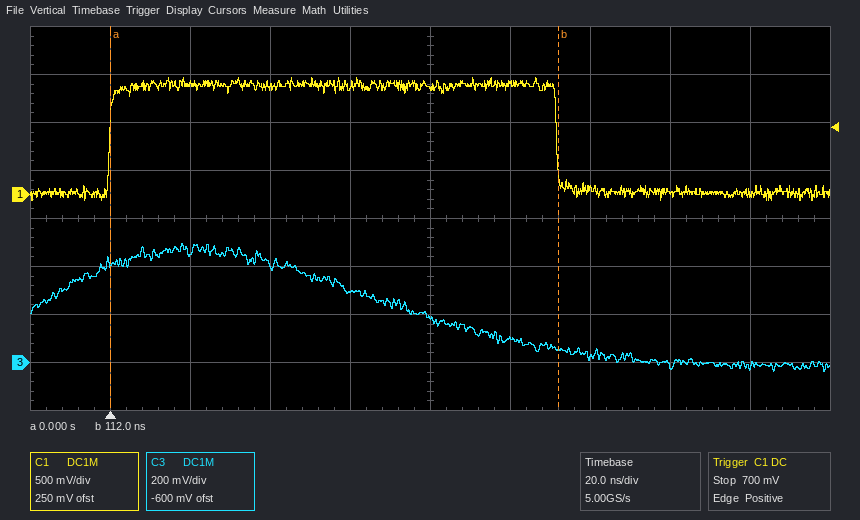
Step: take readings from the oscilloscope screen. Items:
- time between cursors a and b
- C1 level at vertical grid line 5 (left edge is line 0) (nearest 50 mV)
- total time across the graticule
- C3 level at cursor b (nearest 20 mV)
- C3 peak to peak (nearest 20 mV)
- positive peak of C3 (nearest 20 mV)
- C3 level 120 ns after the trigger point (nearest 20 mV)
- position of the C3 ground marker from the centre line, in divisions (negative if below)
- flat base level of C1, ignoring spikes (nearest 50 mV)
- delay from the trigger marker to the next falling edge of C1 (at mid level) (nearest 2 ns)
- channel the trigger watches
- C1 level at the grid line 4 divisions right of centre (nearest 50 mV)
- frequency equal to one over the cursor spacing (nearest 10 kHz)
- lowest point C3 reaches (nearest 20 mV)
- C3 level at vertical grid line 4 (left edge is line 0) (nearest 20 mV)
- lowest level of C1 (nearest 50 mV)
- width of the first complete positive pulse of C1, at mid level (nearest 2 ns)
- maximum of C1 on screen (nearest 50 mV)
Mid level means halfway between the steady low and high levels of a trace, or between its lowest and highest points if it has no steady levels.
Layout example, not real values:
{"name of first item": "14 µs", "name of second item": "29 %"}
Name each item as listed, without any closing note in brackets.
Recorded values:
{"time between cursors a and b": "112 ns", "C1 level at vertical grid line 5 (left edge is line 0)": "1.10 V", "total time across the graticule": "200 ns", "C3 level at cursor b": "60 mV", "C3 peak to peak": "540 mV", "positive peak of C3": "500 mV", "C3 level 120 ns after the trigger point": "20 mV", "position of the C3 ground marker from the centre line, in divisions": "-3.0 div", "flat base level of C1, ignoring spikes": "0 mV", "delay from the trigger marker to the next falling edge of C1 (at mid level)": "112 ns", "channel the trigger watches": "C1", "C1 level at the grid line 4 divisions right of centre": "0 mV", "frequency equal to one over the cursor spacing": "8.93 MHz", "lowest point C3 reaches": "-40 mV", "C3 level at vertical grid line 4 (left edge is line 0)": "300 mV", "lowest level of C1": "-50 mV", "width of the first complete positive pulse of C1, at mid level": "112 ns", "maximum of C1 on screen": "1.20 V"}
